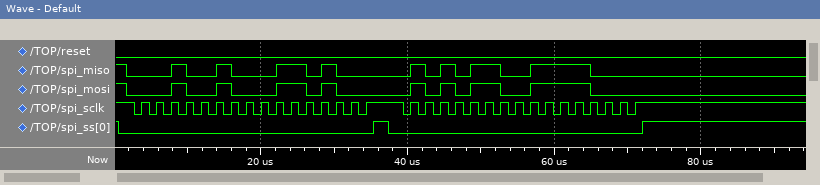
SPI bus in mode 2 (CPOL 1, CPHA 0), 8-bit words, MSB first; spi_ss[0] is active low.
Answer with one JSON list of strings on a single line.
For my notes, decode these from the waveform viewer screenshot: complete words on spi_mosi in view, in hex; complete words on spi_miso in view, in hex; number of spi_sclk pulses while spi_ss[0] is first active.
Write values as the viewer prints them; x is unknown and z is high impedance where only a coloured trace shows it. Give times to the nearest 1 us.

["12, 34, 56, 78", "12, 34, 56, 78", "16"]
